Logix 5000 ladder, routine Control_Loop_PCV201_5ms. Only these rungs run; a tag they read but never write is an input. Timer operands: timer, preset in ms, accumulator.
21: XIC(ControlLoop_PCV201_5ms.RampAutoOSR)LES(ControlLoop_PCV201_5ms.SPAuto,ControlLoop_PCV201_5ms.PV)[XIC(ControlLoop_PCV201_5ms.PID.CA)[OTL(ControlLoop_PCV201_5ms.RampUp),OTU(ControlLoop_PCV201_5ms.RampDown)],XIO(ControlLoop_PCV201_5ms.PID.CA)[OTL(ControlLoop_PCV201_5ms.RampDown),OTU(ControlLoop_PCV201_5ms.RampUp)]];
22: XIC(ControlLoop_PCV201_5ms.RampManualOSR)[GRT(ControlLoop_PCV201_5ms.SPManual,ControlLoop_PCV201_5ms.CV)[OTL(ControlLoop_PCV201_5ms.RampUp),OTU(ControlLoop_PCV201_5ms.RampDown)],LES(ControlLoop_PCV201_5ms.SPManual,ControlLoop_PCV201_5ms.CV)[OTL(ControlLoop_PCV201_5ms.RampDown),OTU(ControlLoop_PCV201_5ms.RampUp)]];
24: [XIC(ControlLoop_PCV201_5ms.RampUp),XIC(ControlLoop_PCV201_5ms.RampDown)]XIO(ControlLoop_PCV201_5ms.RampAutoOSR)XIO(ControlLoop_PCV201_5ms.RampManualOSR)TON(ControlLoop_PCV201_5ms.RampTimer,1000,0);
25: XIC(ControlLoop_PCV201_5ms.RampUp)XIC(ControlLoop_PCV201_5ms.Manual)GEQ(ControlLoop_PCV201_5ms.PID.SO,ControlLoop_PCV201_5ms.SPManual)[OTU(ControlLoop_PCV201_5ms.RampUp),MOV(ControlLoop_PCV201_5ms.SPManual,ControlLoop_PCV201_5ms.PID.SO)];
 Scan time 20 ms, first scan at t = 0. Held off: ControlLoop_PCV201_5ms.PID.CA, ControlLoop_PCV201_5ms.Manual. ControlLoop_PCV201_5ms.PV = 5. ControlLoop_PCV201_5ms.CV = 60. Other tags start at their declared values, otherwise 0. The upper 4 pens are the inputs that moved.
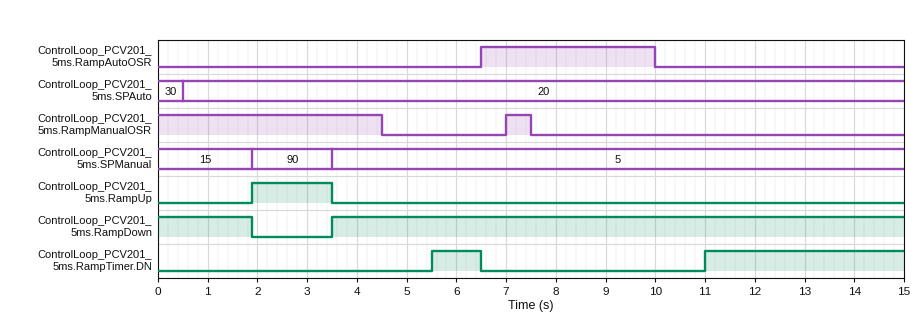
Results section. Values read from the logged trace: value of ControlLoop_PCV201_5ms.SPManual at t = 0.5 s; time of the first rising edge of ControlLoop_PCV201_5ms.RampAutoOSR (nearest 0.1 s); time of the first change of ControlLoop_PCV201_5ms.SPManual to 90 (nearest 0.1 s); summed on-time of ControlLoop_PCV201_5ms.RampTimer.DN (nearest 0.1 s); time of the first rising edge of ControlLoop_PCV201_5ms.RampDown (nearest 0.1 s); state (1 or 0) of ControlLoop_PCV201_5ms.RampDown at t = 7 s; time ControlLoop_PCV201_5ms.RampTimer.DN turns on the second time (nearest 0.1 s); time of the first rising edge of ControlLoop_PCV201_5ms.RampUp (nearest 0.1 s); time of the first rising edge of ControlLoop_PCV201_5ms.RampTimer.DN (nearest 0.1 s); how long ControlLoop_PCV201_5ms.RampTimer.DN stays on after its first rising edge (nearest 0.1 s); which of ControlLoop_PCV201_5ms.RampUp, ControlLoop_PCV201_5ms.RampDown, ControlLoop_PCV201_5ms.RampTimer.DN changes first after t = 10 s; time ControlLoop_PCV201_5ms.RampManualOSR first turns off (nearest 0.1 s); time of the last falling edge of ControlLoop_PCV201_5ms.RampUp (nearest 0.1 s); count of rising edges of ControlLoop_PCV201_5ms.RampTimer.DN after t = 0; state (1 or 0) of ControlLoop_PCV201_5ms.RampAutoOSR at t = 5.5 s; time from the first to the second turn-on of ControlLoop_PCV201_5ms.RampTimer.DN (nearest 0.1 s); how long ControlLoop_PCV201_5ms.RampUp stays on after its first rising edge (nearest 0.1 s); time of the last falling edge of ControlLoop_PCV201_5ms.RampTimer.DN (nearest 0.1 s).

15
6.5 s
1.9 s
5.0 s
3.5 s
1
11.0 s
1.9 s
5.5 s
1.0 s
ControlLoop_PCV201_5ms.RampTimer.DN
4.5 s
3.5 s
2
0
5.5 s
1.6 s
6.5 s
